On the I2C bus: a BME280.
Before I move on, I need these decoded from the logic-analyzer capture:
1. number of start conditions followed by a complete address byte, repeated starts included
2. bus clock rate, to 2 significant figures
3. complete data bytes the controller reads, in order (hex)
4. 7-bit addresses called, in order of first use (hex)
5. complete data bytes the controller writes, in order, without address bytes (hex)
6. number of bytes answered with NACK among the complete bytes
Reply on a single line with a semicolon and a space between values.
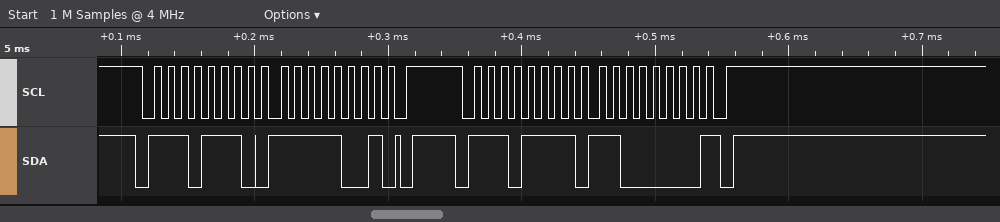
2; 100 kHz; C0; 0x77; F9; 1
